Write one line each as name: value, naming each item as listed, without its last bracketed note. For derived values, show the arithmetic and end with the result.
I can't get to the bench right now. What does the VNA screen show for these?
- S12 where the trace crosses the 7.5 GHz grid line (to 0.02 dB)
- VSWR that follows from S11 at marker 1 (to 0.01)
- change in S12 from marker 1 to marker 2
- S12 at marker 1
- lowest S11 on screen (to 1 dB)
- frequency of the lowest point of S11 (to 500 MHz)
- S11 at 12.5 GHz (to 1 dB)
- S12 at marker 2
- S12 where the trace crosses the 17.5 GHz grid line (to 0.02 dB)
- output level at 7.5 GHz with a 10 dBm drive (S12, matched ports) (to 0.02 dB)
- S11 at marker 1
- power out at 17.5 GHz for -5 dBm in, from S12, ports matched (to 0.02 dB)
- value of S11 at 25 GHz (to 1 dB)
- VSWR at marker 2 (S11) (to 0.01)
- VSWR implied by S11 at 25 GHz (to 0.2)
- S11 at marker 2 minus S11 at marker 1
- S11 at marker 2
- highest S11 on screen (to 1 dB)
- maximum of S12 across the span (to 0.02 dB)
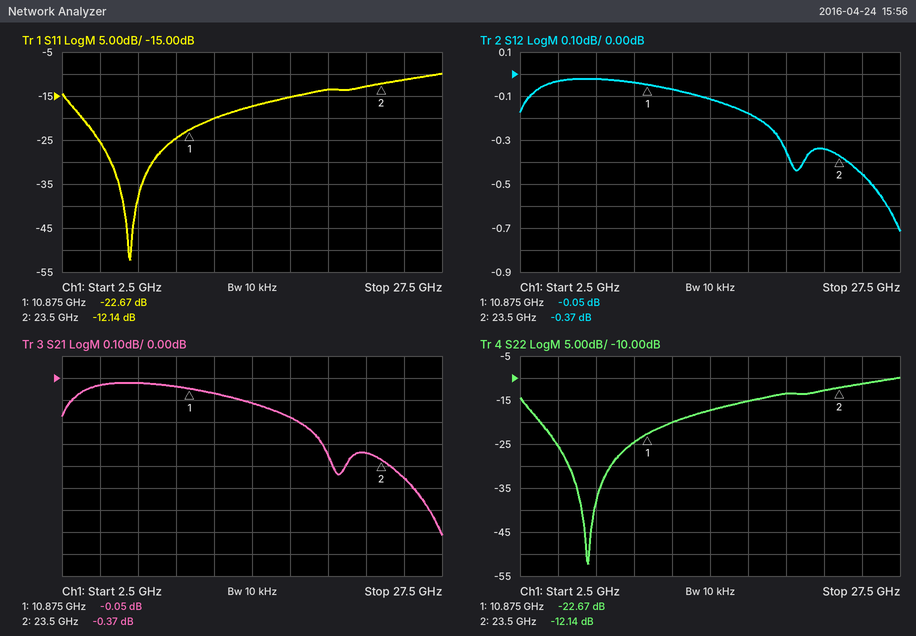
S12 where the trace crosses the 7.5 GHz grid line: -0.02 dB
VSWR that follows from S11 at marker 1: (1 + 0.0735)/(1 − 0.0735) ≈ 1.16
change in S12 from marker 1 to marker 2: -0.37 − (-0.05) = -0.32 dB
S12 at marker 1: -0.05 dB
lowest S11 on screen: -52 dB
frequency of the lowest point of S11: 7.0 GHz
S11 at 12.5 GHz: -20 dB
S12 at marker 2: -0.37 dB
S12 where the trace crosses the 17.5 GHz grid line: -0.18 dB
output level at 7.5 GHz with a 10 dBm drive (S12, matched ports): 10 dBm + (-0.02 dB) = 9.98 dBm
S11 at marker 1: -22.67 dB
power out at 17.5 GHz for -5 dBm in, from S12, ports matched: -5 dBm + (-0.18 dB) = -5.18 dBm
value of S11 at 25 GHz: -11 dB
VSWR at marker 2 (S11): (1 + 0.2472)/(1 − 0.2472) ≈ 1.66
VSWR implied by S11 at 25 GHz: |Γ| = 10^(-11/20) = 0.2818; VSWR = (1 + 0.2818)/(1 − 0.2818) ≈ 1.8
S11 at marker 2 minus S11 at marker 1: -12.14 − (-22.67) = 10.53 dB
S11 at marker 2: -12.14 dB
highest S11 on screen: -10 dB
maximum of S12 across the span: -0.02 dB
